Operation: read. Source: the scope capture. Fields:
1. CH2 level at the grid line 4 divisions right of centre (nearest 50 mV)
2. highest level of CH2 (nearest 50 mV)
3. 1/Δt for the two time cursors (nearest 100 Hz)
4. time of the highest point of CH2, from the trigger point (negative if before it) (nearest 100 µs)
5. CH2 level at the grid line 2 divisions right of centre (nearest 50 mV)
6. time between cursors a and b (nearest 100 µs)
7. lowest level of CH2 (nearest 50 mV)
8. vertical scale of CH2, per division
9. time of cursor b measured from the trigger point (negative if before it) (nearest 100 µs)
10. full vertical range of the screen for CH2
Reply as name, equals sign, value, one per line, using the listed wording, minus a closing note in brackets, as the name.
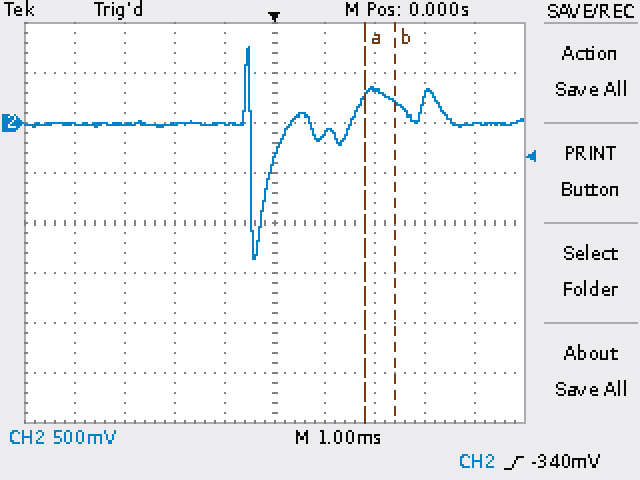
CH2 level at the grid line 4 divisions right of centre = 0 mV
highest level of CH2 = 750 mV
1/Δt for the two time cursors = 1.7 kHz
time of the highest point of CH2, from the trigger point (negative if before it) = -500 µs
CH2 level at the grid line 2 divisions right of centre = 350 mV
time between cursors a and b = 600 µs
lowest level of CH2 = -1.35 V
vertical scale of CH2, per division = 500 mV
time of cursor b measured from the trigger point (negative if before it) = +2.4 ms
full vertical range of the screen for CH2 = 4 V
